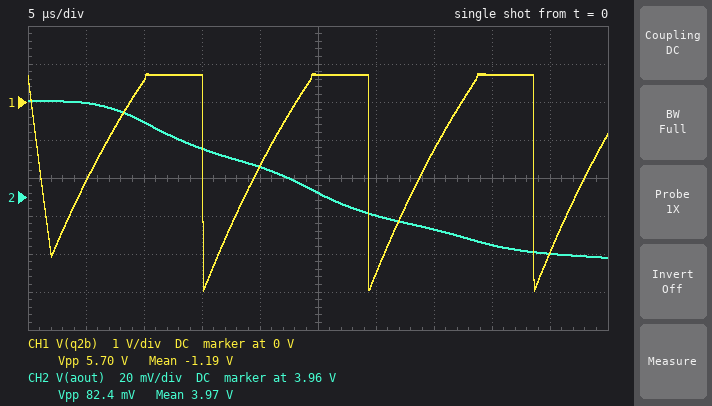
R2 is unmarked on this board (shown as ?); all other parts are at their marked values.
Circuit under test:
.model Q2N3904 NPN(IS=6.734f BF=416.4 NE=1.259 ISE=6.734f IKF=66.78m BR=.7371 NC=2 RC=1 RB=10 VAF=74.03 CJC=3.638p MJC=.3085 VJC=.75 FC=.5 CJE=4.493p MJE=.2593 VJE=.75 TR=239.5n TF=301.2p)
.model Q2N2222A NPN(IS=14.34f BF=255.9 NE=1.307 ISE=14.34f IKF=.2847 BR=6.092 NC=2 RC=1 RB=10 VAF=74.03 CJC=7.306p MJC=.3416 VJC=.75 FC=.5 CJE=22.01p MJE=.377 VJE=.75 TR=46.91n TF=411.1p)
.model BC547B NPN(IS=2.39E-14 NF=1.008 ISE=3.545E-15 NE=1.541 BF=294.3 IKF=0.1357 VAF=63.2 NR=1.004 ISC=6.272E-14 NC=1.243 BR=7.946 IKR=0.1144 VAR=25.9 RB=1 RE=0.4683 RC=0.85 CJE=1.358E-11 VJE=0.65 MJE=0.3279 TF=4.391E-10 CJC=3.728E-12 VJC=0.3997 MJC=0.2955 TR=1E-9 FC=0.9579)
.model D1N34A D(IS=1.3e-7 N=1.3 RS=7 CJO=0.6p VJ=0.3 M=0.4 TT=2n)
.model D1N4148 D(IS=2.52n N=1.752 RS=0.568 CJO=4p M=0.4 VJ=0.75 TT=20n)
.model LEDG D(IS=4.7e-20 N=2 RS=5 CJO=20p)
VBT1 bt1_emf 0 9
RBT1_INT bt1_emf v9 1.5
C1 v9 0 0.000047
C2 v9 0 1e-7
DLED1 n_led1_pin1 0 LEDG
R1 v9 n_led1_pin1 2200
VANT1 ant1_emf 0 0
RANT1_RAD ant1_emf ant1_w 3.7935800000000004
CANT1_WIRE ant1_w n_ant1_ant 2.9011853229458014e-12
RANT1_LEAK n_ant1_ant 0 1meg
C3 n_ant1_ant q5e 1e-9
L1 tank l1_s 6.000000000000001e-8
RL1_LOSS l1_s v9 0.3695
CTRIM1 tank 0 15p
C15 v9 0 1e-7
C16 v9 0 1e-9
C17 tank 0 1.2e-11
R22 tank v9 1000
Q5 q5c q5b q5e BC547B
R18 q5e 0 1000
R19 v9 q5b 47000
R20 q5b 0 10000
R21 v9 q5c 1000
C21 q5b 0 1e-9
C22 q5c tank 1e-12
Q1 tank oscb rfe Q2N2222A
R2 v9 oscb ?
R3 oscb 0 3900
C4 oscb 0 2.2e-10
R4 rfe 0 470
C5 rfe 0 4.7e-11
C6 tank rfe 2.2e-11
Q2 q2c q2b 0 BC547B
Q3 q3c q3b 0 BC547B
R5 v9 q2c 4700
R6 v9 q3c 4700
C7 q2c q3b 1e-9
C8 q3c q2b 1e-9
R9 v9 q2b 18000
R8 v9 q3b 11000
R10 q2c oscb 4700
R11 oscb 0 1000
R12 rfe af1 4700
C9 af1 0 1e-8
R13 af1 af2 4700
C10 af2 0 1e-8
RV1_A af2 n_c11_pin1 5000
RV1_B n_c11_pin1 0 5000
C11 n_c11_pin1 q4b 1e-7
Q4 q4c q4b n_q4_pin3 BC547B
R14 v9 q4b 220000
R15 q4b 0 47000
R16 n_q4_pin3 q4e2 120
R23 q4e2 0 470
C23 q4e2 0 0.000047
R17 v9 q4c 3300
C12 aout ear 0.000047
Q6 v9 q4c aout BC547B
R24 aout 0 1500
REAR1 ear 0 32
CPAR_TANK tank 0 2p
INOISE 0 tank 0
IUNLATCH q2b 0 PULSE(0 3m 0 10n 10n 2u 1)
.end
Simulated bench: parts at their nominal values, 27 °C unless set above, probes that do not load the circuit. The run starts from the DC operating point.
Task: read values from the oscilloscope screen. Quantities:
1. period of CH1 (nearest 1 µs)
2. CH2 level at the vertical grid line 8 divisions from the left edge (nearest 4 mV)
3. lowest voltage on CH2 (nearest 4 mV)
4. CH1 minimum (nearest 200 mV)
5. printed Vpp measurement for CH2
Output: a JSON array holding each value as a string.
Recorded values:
["14 µs", "3.936 V", "3.928 V", "-5.0 V", "82.4 mV"]
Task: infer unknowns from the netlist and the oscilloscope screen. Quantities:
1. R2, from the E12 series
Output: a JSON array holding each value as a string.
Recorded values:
["27 kΩ"]
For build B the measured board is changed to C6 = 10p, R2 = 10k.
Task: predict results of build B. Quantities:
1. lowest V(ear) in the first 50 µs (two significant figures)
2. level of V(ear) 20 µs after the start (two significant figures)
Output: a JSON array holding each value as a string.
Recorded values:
["-84 mV", "-78 mV"]
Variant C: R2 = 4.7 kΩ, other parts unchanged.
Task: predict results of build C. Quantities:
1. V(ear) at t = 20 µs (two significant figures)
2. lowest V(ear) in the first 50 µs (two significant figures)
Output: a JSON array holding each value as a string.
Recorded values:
["-81 mV", "-84 mV"]
